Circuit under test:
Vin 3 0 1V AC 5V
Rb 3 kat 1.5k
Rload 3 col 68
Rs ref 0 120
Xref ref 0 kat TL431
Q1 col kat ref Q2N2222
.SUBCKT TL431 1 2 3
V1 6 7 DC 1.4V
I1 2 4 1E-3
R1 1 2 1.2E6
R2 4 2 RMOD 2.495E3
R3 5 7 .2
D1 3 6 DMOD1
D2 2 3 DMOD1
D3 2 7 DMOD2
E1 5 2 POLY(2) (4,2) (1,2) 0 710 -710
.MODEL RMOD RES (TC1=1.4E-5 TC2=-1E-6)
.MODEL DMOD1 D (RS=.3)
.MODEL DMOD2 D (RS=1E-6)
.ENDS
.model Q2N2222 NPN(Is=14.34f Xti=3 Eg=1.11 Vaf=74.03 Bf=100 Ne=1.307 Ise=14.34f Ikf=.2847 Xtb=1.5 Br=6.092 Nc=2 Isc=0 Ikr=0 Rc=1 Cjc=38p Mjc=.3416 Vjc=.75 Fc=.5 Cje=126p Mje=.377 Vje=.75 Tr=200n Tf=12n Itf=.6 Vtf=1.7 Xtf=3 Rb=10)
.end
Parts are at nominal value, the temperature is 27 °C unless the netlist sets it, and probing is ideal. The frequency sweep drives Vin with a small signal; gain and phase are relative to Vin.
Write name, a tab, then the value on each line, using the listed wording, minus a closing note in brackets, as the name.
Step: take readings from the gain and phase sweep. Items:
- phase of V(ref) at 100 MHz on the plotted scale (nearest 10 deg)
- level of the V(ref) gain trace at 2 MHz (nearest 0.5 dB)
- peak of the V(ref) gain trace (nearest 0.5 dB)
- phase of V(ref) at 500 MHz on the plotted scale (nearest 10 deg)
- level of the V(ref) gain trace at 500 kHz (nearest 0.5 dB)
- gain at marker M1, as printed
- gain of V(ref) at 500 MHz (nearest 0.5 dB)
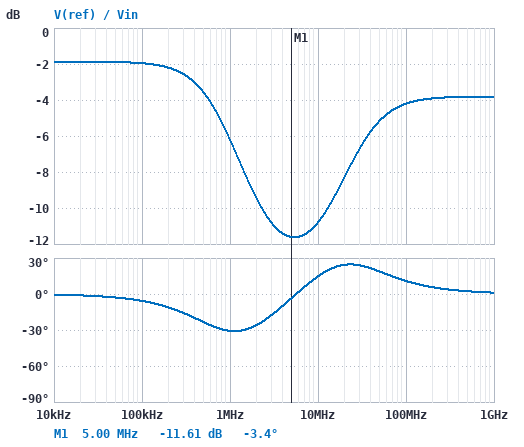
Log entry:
phase of V(ref) at 100 MHz on the plotted scale	10 deg
level of the V(ref) gain trace at 2 MHz	-9.5 dB
peak of the V(ref) gain trace	-2.0 dB
phase of V(ref) at 500 MHz on the plotted scale	0 deg
level of the V(ref) gain trace at 500 kHz	-3.5 dB
gain at marker M1, as printed	-11.61 dB
gain of V(ref) at 500 MHz	-4.0 dB
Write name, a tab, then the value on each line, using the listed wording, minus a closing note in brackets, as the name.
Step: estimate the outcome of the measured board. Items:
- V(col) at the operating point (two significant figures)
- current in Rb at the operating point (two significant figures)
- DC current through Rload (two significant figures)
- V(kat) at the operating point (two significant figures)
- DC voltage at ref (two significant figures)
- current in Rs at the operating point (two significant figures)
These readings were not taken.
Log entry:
V(col) at the operating point	840 mV
current in Rb at the operating point	29 µA
DC current through Rload	2.4 mA
V(kat) at the operating point	960 mV
DC voltage at ref	290 mV
current in Rs at the operating point	2.4 mA
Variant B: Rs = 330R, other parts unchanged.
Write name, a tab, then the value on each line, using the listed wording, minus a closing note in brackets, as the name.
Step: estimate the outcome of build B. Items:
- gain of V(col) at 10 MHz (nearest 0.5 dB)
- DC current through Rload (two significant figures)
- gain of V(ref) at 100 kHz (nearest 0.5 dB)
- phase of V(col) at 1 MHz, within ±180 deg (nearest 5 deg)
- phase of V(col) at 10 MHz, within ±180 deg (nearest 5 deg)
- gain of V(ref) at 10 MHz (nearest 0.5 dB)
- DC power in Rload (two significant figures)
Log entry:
gain of V(col) at 10 MHz	-0.5 dB
DC current through Rload	1.0 mA
gain of V(ref) at 100 kHz	-1.0 dB
phase of V(col) at 1 MHz, within ±180 deg	5 deg
phase of V(col) at 10 MHz, within ±180 deg	0 deg
gain of V(ref) at 10 MHz	-6.0 dB
DC power in Rload	68 µW
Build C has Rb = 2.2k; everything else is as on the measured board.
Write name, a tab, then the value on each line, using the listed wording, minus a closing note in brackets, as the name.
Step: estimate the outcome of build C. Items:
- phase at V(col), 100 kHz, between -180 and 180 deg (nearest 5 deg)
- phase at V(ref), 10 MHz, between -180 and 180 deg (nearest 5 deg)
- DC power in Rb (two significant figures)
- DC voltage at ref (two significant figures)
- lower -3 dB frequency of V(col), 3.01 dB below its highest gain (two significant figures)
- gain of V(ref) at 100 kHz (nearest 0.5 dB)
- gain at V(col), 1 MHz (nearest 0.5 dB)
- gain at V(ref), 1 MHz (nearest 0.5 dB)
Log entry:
phase at V(col), 100 kHz, between -180 and 180 deg	5 deg
phase at V(ref), 10 MHz, between -180 and 180 deg	20 deg
DC power in Rb	1.7 µW
DC voltage at ref	270 mV
lower -3 dB frequency of V(col), 3.01 dB below its highest gain	190 kHz
gain of V(ref) at 100 kHz	-2.5 dB
gain at V(col), 1 MHz	-1.5 dB
gain at V(ref), 1 MHz	-8.0 dB
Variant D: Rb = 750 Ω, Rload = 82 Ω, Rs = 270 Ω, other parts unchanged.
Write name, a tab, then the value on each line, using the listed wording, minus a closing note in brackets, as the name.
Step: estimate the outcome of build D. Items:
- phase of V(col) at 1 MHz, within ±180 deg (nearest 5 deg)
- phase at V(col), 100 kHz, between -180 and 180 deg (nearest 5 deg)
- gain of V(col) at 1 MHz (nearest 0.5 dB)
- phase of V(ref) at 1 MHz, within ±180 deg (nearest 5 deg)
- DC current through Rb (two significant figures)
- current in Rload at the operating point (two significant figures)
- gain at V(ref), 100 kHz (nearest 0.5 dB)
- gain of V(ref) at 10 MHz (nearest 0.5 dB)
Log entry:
phase of V(col) at 1 MHz, within ±180 deg	5 deg
phase at V(col), 100 kHz, between -180 and 180 deg	0 deg
gain of V(col) at 1 MHz	-2.0 dB
phase of V(ref) at 1 MHz, within ±180 deg	-15 deg
DC current through Rb	16 µA
current in Rload at the operating point	1.2 mA
gain at V(ref), 100 kHz	-1.0 dB
gain of V(ref) at 10 MHz	-6.5 dB
